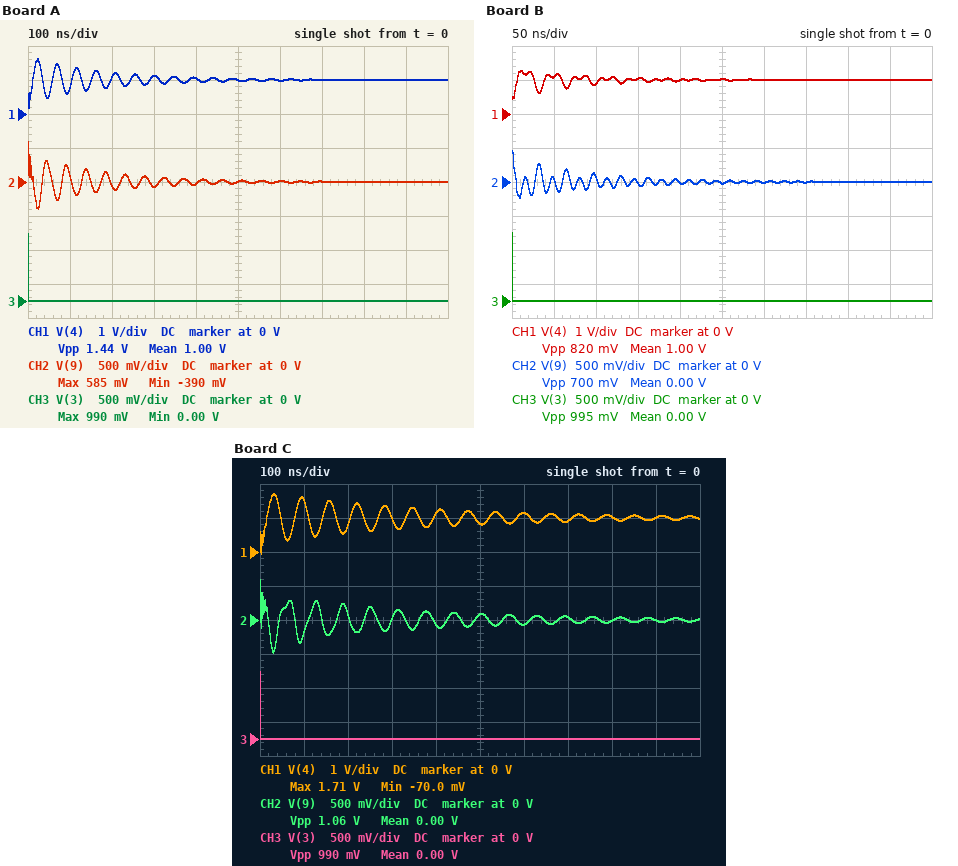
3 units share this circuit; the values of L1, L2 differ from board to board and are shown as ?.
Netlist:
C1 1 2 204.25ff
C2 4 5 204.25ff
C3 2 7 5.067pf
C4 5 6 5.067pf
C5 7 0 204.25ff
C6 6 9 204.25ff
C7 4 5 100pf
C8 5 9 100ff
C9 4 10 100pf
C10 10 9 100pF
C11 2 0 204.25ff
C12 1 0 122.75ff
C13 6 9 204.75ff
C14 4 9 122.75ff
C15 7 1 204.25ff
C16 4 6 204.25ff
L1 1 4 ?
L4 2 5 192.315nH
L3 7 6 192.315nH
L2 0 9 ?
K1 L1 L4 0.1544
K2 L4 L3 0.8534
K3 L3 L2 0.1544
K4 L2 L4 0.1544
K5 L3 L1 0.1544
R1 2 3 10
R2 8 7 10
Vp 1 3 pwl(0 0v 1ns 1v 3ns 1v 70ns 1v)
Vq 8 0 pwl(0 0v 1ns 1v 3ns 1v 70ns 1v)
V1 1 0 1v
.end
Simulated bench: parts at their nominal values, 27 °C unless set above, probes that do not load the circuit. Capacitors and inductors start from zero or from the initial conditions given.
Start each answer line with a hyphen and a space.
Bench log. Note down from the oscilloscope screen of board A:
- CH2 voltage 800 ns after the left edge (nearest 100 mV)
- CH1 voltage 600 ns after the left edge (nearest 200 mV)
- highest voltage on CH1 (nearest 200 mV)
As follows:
- 0 V
- 1.0 V
- 1.6 V
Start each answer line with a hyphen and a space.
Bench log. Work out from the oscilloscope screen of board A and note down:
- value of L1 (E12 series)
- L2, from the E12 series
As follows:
- 270 nH
- 330 nH
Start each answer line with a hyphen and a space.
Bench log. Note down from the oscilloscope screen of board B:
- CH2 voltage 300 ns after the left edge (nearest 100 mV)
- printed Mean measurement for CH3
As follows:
- 0 V
- 0.00 V
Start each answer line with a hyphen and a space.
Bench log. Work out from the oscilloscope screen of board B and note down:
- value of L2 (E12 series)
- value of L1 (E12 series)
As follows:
- 82 nH
- 100 nH
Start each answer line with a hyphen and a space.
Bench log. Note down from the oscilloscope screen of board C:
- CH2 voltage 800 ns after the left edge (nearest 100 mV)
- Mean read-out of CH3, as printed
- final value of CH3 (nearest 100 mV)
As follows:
- 0 V
- 0.00 V
- 0 V
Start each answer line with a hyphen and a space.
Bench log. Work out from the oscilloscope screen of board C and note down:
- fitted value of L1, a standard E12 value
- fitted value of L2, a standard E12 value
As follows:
- 560 nH
- 560 nH
